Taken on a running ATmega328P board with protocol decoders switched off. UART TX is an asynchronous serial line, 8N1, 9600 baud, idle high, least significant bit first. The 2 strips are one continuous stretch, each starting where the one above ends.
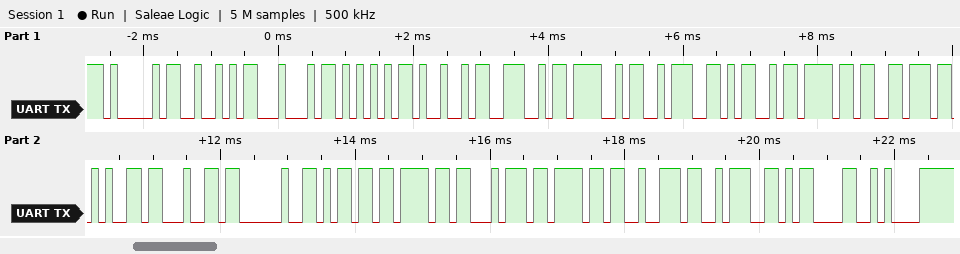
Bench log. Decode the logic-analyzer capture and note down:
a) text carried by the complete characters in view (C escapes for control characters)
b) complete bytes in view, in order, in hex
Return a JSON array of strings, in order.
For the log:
["\"ARDUINO:Moved motor:\\r\\n\"", "41 52 44 55 49 4E 4F 3A 4D 6F 76 65 64 20 6D 6F 74 6F 72 3A 0D 0A"]
